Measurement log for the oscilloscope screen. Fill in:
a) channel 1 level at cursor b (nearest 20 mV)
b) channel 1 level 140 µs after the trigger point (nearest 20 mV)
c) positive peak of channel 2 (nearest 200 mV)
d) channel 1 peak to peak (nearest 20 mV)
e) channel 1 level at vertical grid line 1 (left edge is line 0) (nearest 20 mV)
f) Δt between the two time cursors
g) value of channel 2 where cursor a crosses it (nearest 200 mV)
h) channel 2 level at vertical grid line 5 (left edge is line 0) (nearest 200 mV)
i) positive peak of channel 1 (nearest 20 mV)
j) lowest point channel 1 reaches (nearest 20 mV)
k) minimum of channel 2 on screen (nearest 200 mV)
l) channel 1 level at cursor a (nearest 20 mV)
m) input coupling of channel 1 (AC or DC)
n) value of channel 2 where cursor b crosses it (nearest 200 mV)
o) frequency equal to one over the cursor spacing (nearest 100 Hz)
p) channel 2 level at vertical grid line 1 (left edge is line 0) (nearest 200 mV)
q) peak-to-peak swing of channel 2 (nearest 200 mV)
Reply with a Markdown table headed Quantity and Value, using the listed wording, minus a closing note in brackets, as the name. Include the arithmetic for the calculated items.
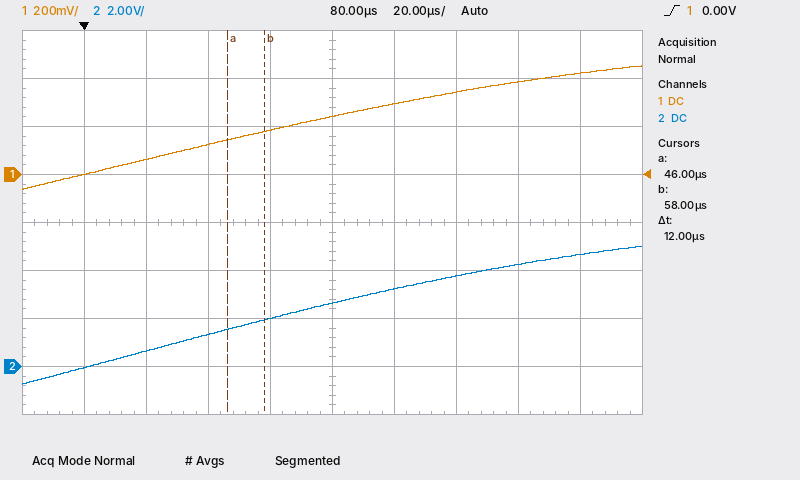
| Quantity | Value |
|---|---|
| channel 1 level at cursor b | 180 mV |
| channel 1 level 140 µs after the trigger point | 380 mV |
| positive peak of channel 2 | 5.0 V |
| channel 1 peak to peak | 460 mV − (-60 mV) = 520 mV |
| channel 1 level at vertical grid line 1 (left edge is line 0) | 0 mV |
| Δt between the two time cursors | 12 µs |
| value of channel 2 where cursor a crosses it | 1.6 V |
| channel 2 level at vertical grid line 5 (left edge is line 0) | 2.6 V |
| positive peak of channel 1 | 460 mV |
| lowest point channel 1 reaches | -60 mV |
| minimum of channel 2 on screen | -800 mV |
| channel 1 level at cursor a | 140 mV |
| input coupling of channel 1 | DC |
| value of channel 2 where cursor b crosses it | 2.0 V |
| frequency equal to one over the cursor spacing | 1 / 12 µs ≈ 83.3 kHz |
| channel 2 level at vertical grid line 1 (left edge is line 0) | 0.0 V |
| peak-to-peak swing of channel 2 | 5.0 V − (-800 mV) = 5.8 V |
